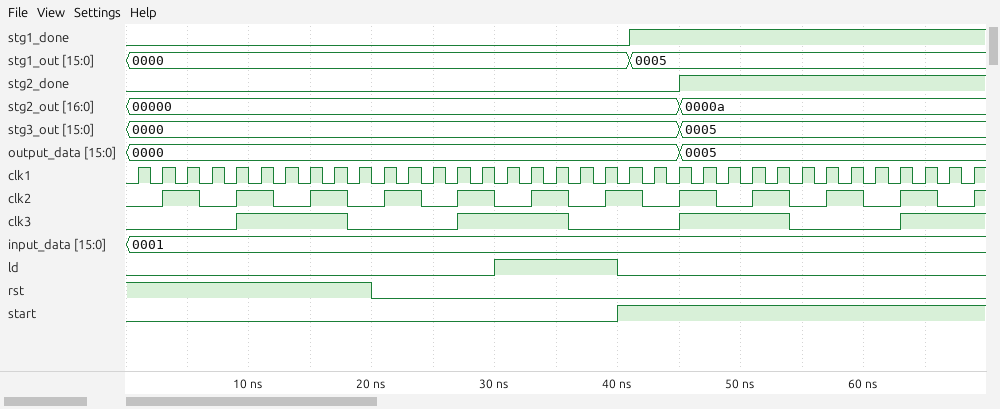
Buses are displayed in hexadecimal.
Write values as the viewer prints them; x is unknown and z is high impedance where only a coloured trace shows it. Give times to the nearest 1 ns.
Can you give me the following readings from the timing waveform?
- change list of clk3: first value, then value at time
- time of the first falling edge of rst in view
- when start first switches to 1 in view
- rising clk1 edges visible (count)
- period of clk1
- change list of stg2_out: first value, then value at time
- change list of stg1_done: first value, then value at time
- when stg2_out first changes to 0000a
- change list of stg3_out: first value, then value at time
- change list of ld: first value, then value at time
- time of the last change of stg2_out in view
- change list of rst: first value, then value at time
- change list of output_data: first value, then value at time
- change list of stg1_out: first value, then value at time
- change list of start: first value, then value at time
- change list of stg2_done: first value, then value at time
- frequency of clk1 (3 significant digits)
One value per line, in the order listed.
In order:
0, 1 at 9 ns, 0 at 18 ns, 1 at 27 ns, 0 at 36 ns, 1 at 45 ns, 0 at 54 ns, 1 at 63 ns
20 ns
40 ns
35
2 ns
00000, 0000a at 45 ns
0, 1 at 41 ns
45 ns
0000, 0005 at 45 ns
0, 1 at 30 ns, 0 at 40 ns
45 ns
1, 0 at 20 ns
0000, 0005 at 45 ns
0000, 0005 at 41 ns
0, 1 at 40 ns
0, 1 at 45 ns
500 MHz
